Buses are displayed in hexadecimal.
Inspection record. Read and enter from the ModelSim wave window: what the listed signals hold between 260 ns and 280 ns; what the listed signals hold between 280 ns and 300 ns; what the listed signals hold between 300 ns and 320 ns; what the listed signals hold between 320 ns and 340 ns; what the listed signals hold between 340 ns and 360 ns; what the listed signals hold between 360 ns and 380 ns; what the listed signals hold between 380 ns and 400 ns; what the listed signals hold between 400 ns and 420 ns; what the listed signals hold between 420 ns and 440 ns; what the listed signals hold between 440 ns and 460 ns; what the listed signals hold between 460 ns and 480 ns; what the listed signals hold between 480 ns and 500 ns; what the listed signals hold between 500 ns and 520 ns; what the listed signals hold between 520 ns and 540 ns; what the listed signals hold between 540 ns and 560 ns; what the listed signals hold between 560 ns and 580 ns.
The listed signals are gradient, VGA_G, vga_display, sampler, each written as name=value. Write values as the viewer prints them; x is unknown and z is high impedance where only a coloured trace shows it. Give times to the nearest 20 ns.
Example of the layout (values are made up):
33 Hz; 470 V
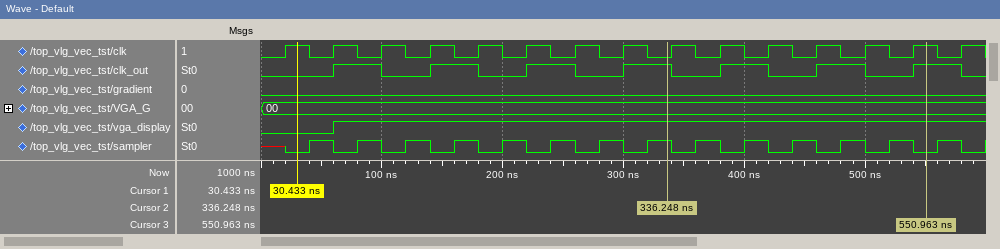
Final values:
gradient=0, VGA_G=00, vga_display=1, sampler=0; gradient=0, VGA_G=00, vga_display=1, sampler=1; gradient=0, VGA_G=00, vga_display=1, sampler=0; gradient=0, VGA_G=00, vga_display=1, sampler=1; gradient=0, VGA_G=00, vga_display=1, sampler=0; gradient=0, VGA_G=00, vga_display=1, sampler=1; gradient=0, VGA_G=00, vga_display=1, sampler=0; gradient=0, VGA_G=00, vga_display=1, sampler=1; gradient=0, VGA_G=00, vga_display=1, sampler=0; gradient=0, VGA_G=00, vga_display=1, sampler=1; gradient=0, VGA_G=00, vga_display=1, sampler=0; gradient=0, VGA_G=00, vga_display=1, sampler=1; gradient=0, VGA_G=00, vga_display=1, sampler=0; gradient=0, VGA_G=00, vga_display=1, sampler=1; gradient=0, VGA_G=00, vga_display=1, sampler=0; gradient=0, VGA_G=00, vga_display=1, sampler=1
